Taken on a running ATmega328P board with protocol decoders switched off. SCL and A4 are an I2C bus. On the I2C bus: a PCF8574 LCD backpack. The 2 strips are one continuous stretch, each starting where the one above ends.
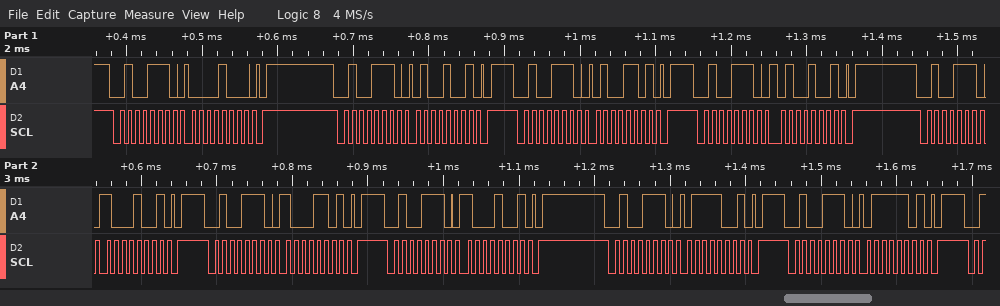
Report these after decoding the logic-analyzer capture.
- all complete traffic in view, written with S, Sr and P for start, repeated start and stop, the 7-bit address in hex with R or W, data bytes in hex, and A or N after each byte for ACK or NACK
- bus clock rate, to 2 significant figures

S 27W A 08 A P S 27W A 49 A P S 27W A 4D A P S 27W A 49 A P S 27W A 89 A P S 27W A 8D A P S 27W A 89 A P S 27W A 79 A P S 27W A 7D A P
100 kHz
